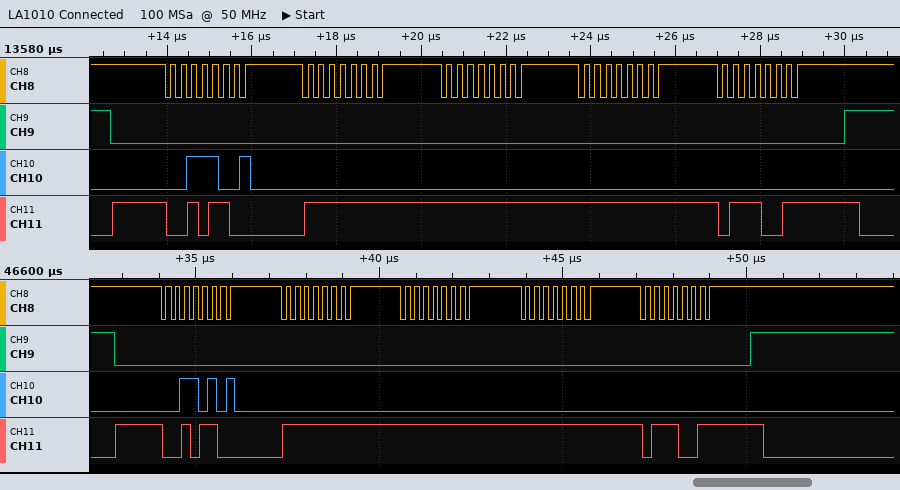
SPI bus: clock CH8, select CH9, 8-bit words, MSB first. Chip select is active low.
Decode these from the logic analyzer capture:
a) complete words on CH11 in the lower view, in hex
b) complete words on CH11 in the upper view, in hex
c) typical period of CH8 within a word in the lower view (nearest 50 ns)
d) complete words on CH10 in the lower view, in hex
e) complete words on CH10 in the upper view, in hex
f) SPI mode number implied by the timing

2C, FF, FF, FF, 73
2C, FF, FF, FF, 73
250 ns
35, 00, 00, 00, 00
39, 00, 00, 00, 00
3
